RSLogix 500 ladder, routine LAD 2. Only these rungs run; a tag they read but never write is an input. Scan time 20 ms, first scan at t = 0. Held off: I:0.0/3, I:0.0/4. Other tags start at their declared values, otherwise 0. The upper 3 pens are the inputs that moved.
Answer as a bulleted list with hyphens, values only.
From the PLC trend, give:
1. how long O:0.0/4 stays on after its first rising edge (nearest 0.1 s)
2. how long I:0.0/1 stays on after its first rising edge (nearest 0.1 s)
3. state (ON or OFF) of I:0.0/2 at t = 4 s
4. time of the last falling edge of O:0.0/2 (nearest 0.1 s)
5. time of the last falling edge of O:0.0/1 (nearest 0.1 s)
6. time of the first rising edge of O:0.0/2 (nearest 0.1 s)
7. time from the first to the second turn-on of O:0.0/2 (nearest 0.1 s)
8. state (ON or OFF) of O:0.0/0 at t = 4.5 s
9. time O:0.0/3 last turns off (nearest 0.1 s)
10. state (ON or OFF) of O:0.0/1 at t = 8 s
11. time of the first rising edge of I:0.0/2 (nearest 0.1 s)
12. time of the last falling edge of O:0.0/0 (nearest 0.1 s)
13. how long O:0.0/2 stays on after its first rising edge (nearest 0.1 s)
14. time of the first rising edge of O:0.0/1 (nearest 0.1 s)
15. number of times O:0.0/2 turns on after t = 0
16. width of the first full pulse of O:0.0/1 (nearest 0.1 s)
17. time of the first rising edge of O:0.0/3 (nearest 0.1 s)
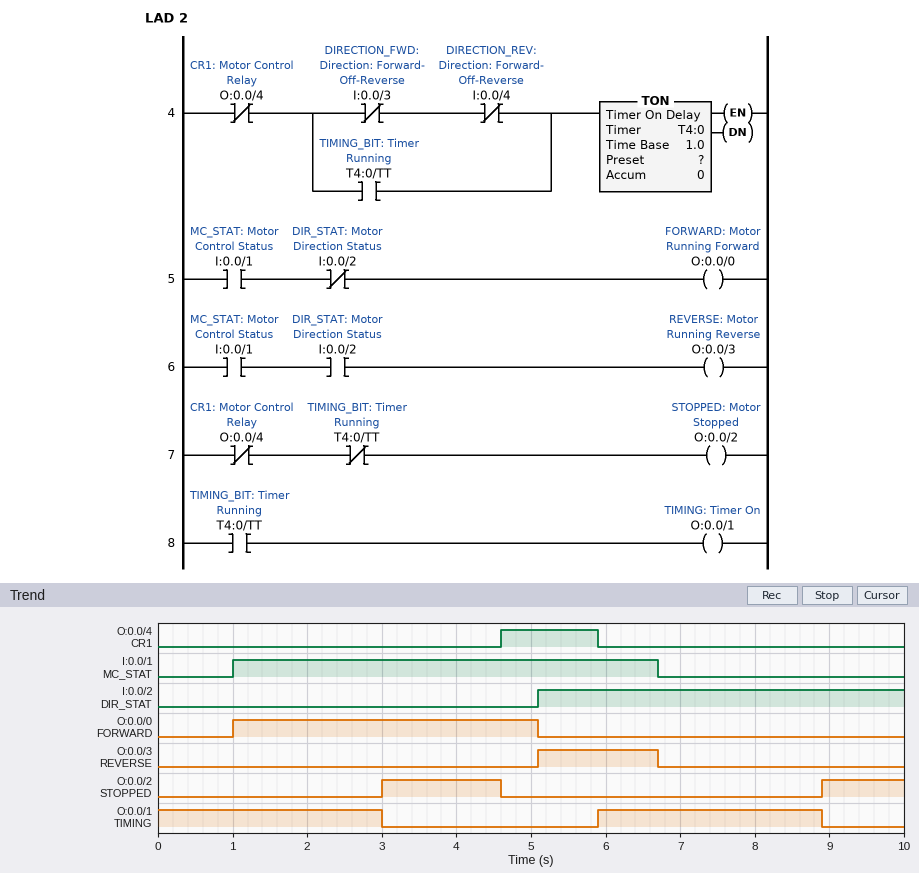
- 1.3 s
- 5.7 s
- OFF
- 4.6 s
- 8.9 s
- 3.0 s
- 5.9 s
- ON
- 6.7 s
- ON
- 5.1 s
- 5.1 s
- 1.6 s
- 5.9 s
- 2
- 3.0 s
- 5.1 s
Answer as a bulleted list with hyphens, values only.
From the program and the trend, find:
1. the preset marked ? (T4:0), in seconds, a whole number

- 3 s
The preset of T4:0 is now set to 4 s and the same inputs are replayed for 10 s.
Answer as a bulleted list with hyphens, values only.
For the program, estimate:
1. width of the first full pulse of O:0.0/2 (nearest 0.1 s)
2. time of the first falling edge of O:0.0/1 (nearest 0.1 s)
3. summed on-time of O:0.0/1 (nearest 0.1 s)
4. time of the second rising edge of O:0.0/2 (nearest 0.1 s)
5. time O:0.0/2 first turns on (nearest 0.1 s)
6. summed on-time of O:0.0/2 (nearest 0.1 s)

- 0.6 s
- 4.0 s
- 8.0 s
- 9.9 s
- 4.0 s
- 0.7 s
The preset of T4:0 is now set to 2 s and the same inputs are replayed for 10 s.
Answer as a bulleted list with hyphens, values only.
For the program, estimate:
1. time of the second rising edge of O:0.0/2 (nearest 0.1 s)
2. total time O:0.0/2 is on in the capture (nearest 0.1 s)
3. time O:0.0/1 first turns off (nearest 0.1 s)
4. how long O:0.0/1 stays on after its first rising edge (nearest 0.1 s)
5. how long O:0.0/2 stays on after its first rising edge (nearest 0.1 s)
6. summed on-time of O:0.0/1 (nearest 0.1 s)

- 7.9 s
- 4.7 s
- 2.0 s
- 2.0 s
- 2.6 s
- 4.0 s
